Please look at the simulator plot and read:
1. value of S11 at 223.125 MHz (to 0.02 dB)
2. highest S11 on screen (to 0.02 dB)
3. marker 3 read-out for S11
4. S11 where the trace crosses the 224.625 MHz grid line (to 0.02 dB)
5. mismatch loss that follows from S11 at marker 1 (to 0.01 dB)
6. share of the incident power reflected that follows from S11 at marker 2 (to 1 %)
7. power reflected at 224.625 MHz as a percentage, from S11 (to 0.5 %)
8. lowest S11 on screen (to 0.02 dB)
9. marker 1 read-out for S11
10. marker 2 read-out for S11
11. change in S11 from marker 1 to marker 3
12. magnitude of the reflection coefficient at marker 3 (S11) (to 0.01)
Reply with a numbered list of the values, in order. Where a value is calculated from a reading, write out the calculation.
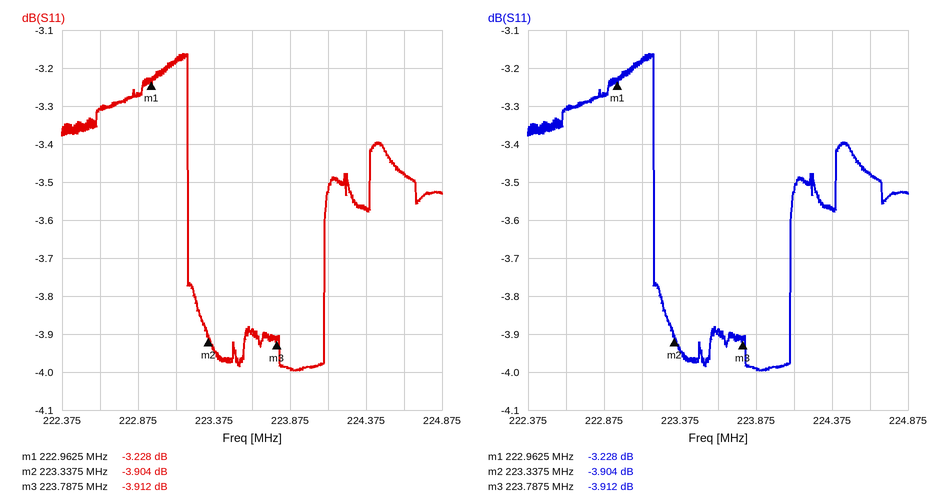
1. -3.18 dB
2. -3.16 dB
3. -3.912 dB
4. -3.48 dB
5. −10 log10(1 − 10^(-3.228/10)) ≈ 2.80 dB
6. 10^(-3.904/10) ≈ 41 %
7. 10^(-3.48/10) ≈ 44.9 %, so 45.0 % to the nearest 0.5 %
8. -4.00 dB
9. -3.228 dB
10. -3.904 dB
11. -3.912 − (-3.228) = -0.684 dB
12. 10^(-3.912/20) ≈ 0.64
